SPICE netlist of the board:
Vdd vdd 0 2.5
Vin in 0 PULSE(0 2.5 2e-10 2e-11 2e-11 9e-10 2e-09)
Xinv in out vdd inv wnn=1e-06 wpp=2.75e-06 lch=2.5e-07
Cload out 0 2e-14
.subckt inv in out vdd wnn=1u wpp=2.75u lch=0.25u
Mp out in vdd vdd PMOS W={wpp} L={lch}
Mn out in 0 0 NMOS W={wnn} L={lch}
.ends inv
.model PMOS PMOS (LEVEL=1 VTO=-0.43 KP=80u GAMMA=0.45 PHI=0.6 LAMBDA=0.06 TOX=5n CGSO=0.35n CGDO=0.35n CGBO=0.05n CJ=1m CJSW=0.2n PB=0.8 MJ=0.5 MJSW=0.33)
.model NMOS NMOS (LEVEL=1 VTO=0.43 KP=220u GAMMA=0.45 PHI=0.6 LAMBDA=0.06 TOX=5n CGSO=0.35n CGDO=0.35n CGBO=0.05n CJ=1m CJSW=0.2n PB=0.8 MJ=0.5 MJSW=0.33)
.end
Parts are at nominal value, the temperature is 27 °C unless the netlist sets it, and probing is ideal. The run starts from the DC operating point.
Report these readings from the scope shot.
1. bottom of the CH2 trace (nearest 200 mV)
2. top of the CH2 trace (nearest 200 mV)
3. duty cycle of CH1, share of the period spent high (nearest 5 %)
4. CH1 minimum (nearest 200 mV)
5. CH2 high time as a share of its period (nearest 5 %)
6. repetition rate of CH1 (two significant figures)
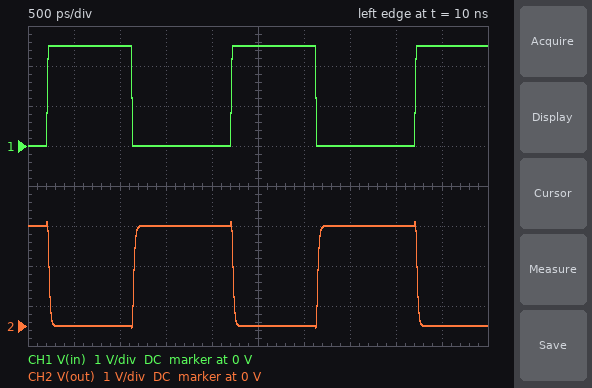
0 V
2.6 V
45 %
0 V
55 %
500 MHz
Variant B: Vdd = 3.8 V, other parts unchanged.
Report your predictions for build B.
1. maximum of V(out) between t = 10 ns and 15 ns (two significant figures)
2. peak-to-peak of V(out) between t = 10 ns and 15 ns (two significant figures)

3.9 V
3.7 V
